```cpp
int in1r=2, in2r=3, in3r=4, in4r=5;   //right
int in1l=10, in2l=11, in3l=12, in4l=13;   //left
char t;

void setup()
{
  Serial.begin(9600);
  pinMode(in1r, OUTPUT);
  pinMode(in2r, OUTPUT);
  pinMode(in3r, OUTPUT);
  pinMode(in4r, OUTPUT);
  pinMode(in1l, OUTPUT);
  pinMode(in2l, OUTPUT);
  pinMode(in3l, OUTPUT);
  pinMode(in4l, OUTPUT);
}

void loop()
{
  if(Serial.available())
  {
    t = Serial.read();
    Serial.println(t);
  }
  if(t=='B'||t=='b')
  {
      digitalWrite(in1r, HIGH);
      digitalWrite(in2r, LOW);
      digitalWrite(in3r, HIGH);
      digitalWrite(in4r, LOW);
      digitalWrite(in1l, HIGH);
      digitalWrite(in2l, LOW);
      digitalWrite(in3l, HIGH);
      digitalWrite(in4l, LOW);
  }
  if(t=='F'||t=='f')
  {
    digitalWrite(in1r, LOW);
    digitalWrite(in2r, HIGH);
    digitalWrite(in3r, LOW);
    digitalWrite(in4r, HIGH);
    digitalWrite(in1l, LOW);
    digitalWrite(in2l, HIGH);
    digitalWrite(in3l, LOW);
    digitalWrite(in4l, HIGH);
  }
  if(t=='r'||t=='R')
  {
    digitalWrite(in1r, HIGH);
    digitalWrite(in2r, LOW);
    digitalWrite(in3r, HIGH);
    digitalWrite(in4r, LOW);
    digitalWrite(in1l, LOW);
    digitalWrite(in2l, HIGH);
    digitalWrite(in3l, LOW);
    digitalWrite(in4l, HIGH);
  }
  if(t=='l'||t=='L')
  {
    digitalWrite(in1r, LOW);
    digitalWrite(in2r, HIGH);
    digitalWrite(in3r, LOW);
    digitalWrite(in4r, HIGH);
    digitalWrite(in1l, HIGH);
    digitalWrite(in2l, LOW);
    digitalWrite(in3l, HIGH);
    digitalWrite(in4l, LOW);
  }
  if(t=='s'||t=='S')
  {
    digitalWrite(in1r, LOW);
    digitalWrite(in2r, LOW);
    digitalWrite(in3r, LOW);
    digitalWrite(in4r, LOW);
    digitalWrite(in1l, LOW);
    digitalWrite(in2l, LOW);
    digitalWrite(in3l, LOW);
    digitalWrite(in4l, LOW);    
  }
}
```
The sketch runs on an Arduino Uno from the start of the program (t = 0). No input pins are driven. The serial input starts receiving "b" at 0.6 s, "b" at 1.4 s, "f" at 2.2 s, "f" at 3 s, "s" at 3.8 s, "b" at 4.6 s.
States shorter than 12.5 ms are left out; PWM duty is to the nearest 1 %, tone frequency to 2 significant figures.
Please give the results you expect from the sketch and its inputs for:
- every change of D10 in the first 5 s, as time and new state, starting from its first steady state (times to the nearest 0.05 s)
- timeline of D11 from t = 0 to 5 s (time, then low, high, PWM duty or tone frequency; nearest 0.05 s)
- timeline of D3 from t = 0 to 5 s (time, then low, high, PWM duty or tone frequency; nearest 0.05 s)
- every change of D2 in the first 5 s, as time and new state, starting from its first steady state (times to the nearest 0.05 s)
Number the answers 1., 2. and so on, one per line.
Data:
1. 0 s low; 0.6 s high; 2.2 s low; 4.6 s high
2. 0 s low; 2.2 s high; 3.8 s low
3. 0 s low; 2.2 s high; 3.8 s low
4. 0 s low; 0.6 s high; 2.2 s low; 4.6 s high
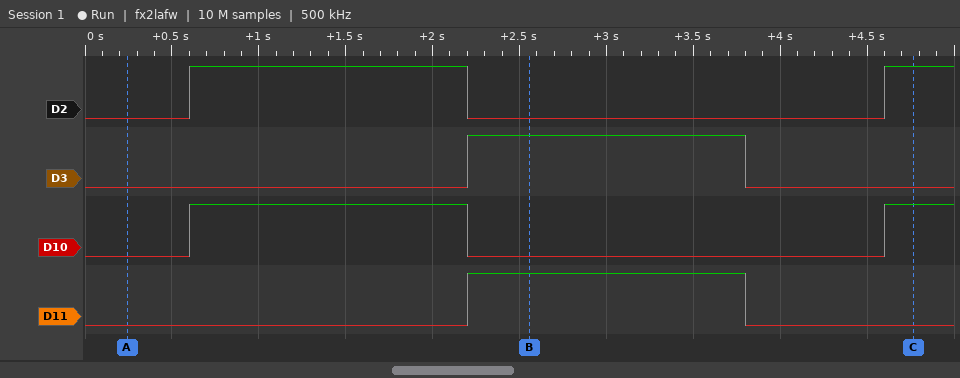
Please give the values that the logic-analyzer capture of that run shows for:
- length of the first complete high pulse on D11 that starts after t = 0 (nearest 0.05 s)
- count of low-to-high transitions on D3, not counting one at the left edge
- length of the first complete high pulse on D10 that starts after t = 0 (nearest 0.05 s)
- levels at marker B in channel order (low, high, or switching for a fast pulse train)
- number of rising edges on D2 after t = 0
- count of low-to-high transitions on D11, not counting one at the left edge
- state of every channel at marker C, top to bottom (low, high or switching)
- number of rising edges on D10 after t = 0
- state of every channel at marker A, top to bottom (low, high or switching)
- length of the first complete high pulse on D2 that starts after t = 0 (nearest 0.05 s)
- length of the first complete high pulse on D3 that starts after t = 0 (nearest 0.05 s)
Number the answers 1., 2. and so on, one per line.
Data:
1. 1.60 s
2. 1
3. 1.60 s
4. D2 low, D3 high, D10 low, D11 high
5. 2
6. 1
7. D2 high, D3 low, D10 high, D11 low
8. 2
9. D2 low, D3 low, D10 low, D11 low
10. 1.60 s
11. 1.60 s
